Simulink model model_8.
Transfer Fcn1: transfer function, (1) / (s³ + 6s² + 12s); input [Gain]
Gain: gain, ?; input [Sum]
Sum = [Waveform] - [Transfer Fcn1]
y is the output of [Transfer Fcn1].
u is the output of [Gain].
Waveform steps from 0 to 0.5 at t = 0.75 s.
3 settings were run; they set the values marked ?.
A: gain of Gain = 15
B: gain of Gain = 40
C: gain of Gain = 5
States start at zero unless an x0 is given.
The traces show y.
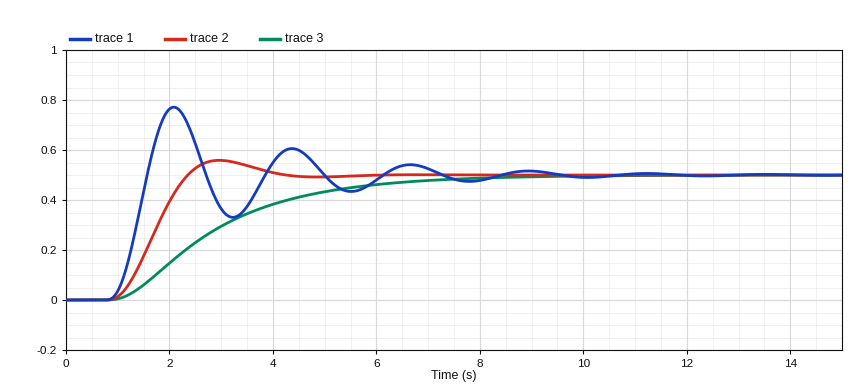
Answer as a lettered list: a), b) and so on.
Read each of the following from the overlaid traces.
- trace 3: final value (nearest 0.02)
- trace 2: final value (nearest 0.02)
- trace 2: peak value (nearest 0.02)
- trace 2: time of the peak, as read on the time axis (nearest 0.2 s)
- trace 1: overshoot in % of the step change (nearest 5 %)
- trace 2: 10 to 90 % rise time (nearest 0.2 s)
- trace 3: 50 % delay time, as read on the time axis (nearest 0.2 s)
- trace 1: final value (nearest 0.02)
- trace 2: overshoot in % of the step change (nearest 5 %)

a) 0.50
b) 0.50
c) 0.56
d) 3.0 s
e) 55 %
f) 1.0 s
g) 2.6 s
h) 0.50
i) 10 %
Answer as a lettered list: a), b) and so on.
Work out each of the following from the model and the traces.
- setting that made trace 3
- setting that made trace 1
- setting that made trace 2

a) C
b) B
c) A
